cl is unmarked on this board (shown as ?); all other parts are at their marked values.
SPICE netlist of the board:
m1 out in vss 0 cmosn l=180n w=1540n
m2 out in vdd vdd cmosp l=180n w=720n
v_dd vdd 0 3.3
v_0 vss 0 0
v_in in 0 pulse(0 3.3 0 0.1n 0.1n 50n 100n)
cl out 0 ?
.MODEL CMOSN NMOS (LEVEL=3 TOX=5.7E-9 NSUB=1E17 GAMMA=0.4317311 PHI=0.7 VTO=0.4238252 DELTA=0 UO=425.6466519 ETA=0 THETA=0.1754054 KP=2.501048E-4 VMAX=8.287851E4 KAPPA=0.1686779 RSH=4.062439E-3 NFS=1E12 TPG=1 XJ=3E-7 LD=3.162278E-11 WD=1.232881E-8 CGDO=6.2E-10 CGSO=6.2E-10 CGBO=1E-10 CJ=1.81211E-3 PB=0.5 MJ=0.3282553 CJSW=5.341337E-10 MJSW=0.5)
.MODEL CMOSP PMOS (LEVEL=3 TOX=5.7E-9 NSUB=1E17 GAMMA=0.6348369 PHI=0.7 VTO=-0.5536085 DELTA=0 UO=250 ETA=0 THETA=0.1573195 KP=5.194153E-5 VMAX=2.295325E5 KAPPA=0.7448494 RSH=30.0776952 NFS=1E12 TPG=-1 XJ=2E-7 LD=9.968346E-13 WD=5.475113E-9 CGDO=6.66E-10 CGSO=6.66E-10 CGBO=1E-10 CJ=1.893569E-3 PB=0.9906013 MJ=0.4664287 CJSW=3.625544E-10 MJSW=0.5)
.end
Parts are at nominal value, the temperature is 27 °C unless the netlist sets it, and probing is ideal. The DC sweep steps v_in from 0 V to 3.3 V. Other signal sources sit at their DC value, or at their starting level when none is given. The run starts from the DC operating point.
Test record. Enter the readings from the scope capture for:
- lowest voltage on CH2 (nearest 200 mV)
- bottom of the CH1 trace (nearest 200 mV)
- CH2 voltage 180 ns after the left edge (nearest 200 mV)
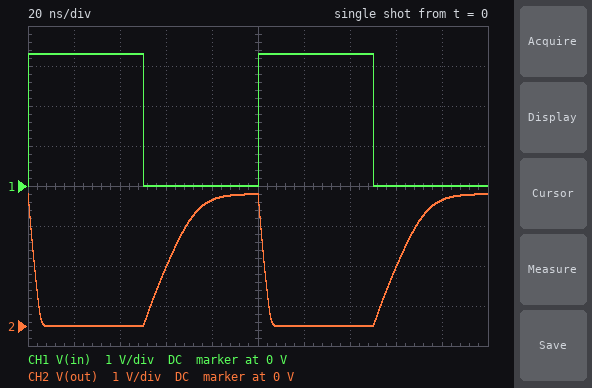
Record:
0 V
0 V
3.2 V
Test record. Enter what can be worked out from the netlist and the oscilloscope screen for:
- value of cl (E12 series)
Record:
2.2 pF
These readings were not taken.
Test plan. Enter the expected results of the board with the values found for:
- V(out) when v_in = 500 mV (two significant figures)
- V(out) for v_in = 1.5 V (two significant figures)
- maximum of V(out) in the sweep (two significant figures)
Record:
3.1 V
85 mV
3.3 V
